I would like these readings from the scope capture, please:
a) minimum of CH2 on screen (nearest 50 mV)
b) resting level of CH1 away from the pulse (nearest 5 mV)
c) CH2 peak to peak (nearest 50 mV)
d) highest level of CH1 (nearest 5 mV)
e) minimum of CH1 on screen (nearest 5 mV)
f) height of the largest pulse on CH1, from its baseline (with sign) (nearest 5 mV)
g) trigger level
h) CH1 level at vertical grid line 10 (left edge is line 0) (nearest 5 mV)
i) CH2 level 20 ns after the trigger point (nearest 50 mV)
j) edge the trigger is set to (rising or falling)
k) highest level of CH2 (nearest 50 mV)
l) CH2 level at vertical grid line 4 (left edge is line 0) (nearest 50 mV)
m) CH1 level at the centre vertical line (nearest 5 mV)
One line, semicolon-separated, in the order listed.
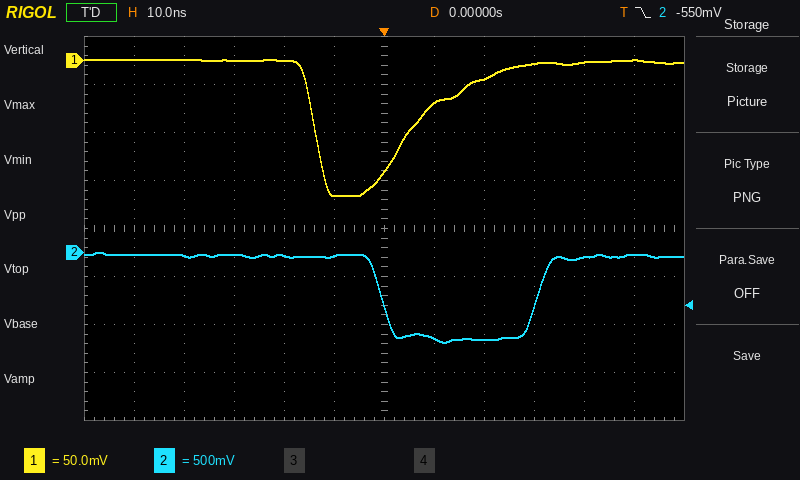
-950 mV; 0 mV; 950 mV; 0 mV; -140 mV; -140 mV; -550 mV; 0 mV; -900 mV; falling; 0 mV; -50 mV; -115 mV
